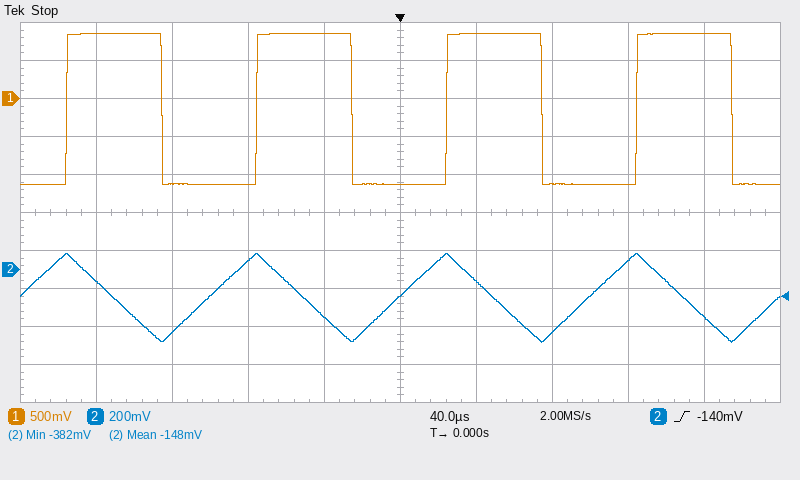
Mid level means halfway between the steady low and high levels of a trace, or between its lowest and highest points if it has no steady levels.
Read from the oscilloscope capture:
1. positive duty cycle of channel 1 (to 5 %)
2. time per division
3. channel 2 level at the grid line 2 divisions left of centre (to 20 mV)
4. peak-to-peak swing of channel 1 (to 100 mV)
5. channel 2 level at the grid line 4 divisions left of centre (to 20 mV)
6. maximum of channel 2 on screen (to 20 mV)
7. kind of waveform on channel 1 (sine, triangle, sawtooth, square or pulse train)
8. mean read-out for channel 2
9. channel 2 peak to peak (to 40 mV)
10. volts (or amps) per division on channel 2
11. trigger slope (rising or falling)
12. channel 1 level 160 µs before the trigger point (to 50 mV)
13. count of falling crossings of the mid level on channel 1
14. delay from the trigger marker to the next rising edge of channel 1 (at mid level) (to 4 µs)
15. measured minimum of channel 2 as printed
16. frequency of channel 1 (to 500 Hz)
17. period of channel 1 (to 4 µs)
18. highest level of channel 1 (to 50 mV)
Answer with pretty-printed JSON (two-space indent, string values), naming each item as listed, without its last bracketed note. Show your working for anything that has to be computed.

{
  "positive duty cycle of channel 1": "50 %",
  "time per division": "40 µs",
  "channel 2 level at the grid line 2 divisions left of centre": "40 mV",
  "peak-to-peak swing of channel 1": "2.00 V",
  "channel 2 level at the grid line 4 divisions left of centre": "-60 mV",
  "maximum of channel 2 on screen": "80 mV",
  "kind of waveform on channel 1": "square",
  "mean read-out for channel 2": "-148 mV",
  "channel 2 peak to peak": "480 mV",
  "volts (or amps) per division on channel 2": "200 mV",
  "trigger slope": "rising",
  "channel 1 level 160 µs before the trigger point": "850 mV",
  "count of falling crossings of the mid level on channel 1": "4",
  "delay from the trigger marker to the next rising edge of channel 1 (at mid level)": "24 µs",
  "measured minimum of channel 2 as printed": "-382 mV",
  "frequency of channel 1": "1 / 100 µs ≈ 10.0 kHz",
  "period of channel 1": "100 µs",
  "highest level of channel 1": "850 mV"
}
